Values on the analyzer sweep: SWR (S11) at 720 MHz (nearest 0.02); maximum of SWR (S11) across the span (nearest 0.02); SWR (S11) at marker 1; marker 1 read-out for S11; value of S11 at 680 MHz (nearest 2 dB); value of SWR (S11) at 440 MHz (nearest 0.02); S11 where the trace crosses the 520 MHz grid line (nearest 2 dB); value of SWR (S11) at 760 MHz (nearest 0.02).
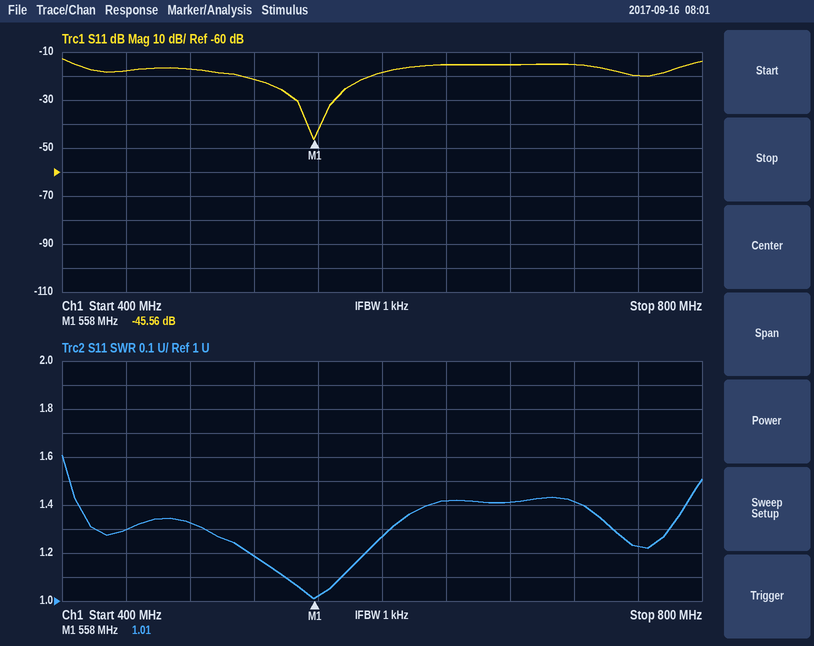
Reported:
1.42
1.60
1.01
-45.56 dB
-16 dB
1.30
-22 dB
1.22
